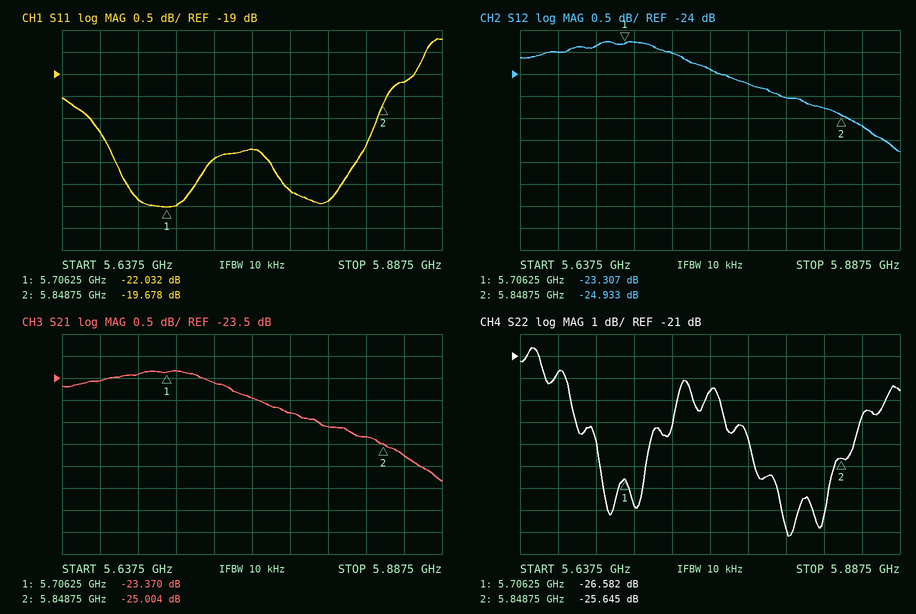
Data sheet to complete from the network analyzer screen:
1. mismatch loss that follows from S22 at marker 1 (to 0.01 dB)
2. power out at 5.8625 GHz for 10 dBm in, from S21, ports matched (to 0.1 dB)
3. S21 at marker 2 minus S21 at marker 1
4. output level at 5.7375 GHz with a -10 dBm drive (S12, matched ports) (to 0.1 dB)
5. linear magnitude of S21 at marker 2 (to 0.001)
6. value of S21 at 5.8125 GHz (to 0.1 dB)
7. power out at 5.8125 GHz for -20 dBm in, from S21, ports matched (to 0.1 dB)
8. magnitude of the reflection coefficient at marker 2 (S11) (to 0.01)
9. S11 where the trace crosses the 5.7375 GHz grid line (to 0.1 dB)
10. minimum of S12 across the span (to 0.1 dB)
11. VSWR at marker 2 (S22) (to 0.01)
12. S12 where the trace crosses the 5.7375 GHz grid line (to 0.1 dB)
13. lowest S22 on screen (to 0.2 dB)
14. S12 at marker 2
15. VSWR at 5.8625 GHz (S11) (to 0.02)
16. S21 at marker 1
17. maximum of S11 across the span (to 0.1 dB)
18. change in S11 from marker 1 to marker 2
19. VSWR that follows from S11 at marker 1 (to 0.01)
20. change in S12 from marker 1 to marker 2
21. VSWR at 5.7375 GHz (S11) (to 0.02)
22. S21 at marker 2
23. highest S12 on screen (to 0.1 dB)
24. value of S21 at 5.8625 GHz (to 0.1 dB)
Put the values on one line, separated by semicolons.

0.01 dB; -15.3 dBm; -1.634 dB; -33.5 dBm; 0.056; -24.6 dB; -44.6 dBm; 0.10; -20.9 dB; -25.8 dB; 1.11; -23.5 dB; -29.2 dB; -24.933 dB; 1.24; -23.370 dB; -18.2 dB; 2.354 dB; 1.17; -1.626 dB; 1.20; -25.004 dB; -23.3 dB; -25.3 dB
